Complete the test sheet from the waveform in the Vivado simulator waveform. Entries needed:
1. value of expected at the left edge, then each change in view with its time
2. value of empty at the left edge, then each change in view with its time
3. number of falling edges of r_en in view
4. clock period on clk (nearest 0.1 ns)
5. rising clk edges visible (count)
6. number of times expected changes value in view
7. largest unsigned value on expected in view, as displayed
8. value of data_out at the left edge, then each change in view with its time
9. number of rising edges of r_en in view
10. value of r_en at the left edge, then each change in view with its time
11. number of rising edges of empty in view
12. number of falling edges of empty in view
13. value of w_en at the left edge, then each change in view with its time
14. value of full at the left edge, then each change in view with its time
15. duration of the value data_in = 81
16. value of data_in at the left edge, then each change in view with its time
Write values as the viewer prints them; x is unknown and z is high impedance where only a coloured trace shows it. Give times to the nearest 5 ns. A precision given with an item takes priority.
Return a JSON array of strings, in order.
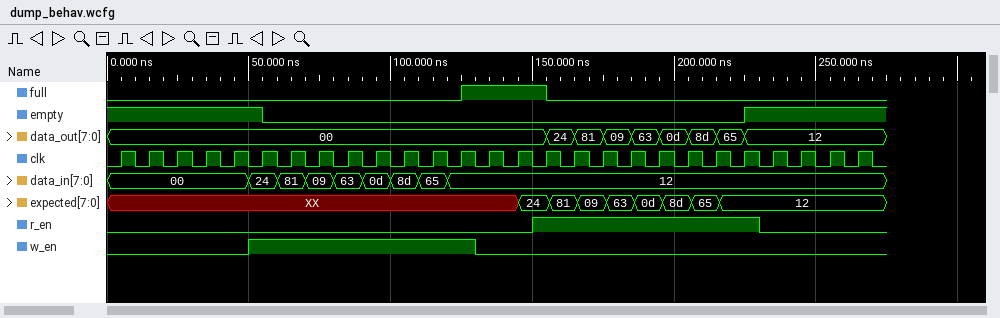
["XX, 24 at 145 ns, 81 at 155 ns, 09 at 165 ns, 63 at 175 ns, 0d at 185 ns, 8d at 195 ns, 65 at 205 ns, 12 at 215 ns", "1, 0 at 55 ns, 1 at 225 ns", "1", "10 ns", "27", "8", "8d", "00, 24 at 155 ns, 81 at 165 ns, 09 at 175 ns, 63 at 185 ns, 0d at 195 ns, 8d at 205 ns, 65 at 215 ns, 12 at 225 ns", "1", "0, 1 at 150 ns, 0 at 230 ns", "1", "1", "0, 1 at 50 ns, 0 at 130 ns", "0, 1 at 125 ns, 0 at 155 ns", "10 ns", "00, 24 at 50 ns, 81 at 60 ns, 09 at 70 ns, 63 at 80 ns, 0d at 90 ns, 8d at 100 ns, 65 at 110 ns, 12 at 120 ns"]
